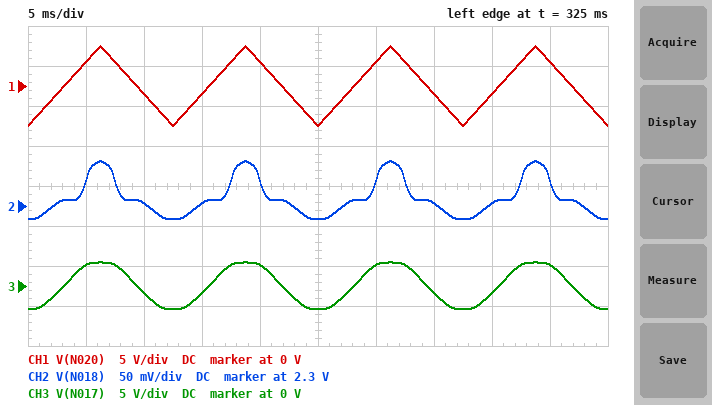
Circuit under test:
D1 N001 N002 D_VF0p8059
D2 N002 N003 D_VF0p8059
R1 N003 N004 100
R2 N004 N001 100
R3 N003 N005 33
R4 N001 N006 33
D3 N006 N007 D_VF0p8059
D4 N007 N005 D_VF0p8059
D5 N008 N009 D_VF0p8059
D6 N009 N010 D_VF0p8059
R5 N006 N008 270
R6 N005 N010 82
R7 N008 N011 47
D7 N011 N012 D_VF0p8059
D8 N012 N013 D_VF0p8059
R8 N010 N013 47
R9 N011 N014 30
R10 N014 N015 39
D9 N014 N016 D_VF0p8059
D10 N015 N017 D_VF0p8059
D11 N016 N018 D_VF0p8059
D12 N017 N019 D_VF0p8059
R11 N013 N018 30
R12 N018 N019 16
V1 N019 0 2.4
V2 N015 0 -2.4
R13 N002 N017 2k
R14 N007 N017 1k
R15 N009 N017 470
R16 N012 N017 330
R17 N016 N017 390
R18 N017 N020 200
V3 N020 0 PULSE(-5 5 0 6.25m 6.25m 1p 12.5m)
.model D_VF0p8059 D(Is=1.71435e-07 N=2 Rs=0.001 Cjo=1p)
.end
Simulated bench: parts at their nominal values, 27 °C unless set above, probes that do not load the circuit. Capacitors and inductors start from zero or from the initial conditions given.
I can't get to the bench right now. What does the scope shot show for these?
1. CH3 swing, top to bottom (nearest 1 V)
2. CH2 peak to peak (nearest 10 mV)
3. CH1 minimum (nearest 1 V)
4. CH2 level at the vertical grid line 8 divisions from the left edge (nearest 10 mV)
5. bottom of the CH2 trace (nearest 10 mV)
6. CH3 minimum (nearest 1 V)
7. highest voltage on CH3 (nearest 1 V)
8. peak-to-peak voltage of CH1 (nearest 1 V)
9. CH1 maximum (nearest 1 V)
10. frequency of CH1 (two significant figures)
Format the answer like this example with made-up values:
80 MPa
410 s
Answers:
6 V
70 mV
-5 V
2.30 V
2.28 V
-3 V
3 V
10 V
5 V
80 Hz
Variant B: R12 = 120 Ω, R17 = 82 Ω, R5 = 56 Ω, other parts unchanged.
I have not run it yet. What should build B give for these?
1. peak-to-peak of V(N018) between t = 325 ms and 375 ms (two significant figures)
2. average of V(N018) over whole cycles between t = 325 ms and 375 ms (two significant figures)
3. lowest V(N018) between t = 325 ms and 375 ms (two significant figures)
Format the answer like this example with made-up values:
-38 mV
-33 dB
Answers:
700 mV
1.7 V
1.5 V
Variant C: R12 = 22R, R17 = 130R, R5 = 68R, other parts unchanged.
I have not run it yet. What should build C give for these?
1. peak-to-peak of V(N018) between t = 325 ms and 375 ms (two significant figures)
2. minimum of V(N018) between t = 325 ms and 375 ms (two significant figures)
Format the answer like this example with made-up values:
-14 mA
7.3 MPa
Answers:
110 mV
2.2 V
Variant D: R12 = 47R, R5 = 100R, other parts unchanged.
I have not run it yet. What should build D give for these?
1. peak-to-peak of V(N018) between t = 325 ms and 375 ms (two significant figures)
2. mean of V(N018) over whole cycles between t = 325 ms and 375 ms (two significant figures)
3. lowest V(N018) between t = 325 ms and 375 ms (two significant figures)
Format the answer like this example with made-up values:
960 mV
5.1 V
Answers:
220 mV
2.1 V
2.0 V
